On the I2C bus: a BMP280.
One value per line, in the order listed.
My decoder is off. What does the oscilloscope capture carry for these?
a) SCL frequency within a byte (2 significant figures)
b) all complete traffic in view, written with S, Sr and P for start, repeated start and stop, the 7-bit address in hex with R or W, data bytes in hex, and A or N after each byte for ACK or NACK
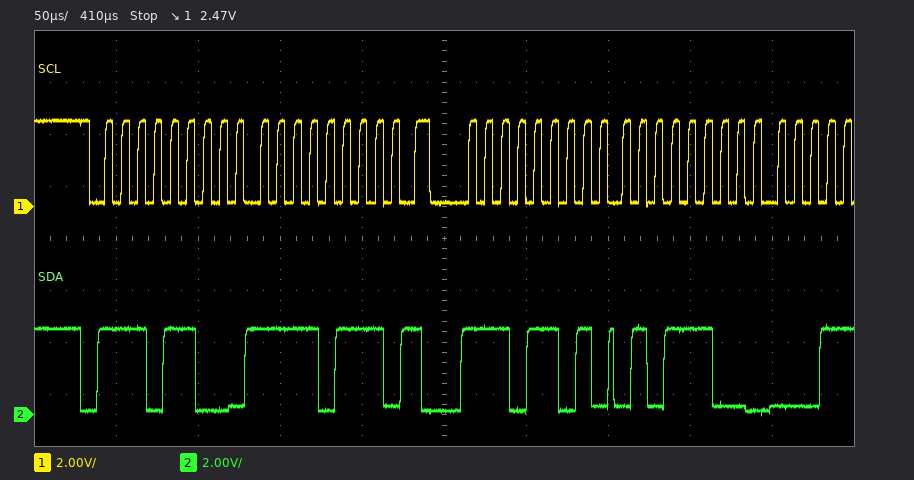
100 kHz
S 76W A F7 A Sr 76R A 5C A
